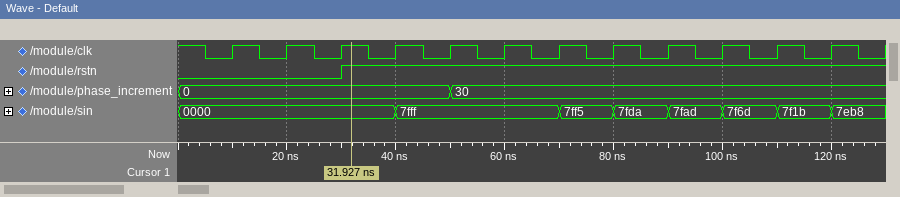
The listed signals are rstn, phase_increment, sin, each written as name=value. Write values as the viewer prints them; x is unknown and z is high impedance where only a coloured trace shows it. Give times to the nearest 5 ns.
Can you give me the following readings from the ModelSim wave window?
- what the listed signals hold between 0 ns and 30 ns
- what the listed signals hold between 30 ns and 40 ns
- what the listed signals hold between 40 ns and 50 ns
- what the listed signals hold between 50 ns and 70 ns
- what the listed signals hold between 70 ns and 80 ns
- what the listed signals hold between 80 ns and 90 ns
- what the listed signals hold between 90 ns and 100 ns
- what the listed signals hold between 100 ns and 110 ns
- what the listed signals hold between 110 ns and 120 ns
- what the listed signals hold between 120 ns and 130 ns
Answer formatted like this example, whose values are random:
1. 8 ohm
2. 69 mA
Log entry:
1. rstn=0, phase_increment=0, sin=0000
2. rstn=1, phase_increment=0, sin=0000
3. rstn=1, phase_increment=0, sin=7fff
4. rstn=1, phase_increment=30, sin=7fff
5. rstn=1, phase_increment=30, sin=7ff5
6. rstn=1, phase_increment=30, sin=7fda
7. rstn=1, phase_increment=30, sin=7fad
8. rstn=1, phase_increment=30, sin=7f6d
9. rstn=1, phase_increment=30, sin=7f1b
10. rstn=1, phase_increment=30, sin=7eb8
